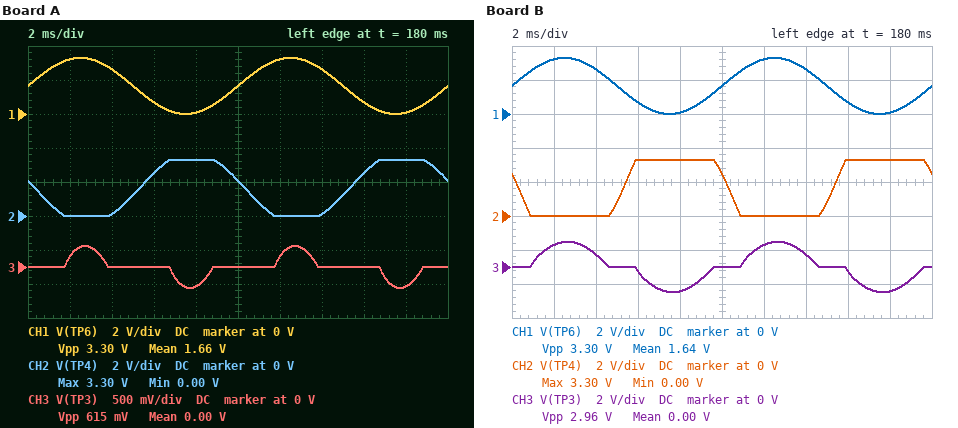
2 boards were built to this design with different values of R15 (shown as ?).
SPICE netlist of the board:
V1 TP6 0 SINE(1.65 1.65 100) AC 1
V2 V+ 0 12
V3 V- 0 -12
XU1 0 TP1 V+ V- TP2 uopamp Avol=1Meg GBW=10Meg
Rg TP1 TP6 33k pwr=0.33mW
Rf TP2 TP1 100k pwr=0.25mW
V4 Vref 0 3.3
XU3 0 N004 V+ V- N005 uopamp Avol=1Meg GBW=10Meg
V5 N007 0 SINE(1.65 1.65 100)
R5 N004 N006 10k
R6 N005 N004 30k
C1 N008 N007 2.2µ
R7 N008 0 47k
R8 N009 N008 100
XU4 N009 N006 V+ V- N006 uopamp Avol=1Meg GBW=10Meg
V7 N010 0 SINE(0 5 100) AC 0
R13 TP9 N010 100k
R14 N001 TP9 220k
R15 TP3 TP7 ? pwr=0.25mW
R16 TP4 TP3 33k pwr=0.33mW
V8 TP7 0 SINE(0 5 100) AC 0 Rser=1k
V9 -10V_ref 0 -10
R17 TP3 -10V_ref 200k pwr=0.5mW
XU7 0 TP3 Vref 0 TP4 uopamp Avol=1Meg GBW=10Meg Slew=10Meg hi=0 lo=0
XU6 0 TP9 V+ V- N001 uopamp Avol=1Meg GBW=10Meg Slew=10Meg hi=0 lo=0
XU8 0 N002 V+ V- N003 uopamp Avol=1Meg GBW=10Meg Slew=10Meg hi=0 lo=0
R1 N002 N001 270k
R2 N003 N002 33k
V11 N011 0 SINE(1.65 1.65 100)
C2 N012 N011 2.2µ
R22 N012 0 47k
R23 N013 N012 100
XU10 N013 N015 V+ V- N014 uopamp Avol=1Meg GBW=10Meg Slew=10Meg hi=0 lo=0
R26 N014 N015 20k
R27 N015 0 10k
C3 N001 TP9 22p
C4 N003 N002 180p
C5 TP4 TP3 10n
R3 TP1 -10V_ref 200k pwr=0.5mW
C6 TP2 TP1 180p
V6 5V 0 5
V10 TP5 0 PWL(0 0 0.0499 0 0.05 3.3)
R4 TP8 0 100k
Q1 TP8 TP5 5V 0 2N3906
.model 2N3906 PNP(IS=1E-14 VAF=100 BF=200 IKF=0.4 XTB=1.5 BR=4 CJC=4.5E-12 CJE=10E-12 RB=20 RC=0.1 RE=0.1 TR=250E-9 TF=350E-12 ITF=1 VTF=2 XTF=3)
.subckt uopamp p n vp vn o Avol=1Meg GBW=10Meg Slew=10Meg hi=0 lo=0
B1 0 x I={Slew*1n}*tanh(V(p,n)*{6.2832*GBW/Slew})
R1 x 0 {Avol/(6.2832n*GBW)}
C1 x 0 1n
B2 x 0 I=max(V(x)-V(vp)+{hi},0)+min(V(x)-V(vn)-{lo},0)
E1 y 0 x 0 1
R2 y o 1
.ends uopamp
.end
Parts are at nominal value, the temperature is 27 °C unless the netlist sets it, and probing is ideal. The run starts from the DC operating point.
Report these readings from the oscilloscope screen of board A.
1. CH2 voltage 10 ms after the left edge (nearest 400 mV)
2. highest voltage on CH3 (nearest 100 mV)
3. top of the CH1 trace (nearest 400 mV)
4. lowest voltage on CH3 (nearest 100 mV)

2.0 V
300 mV
3.2 V
-300 mV
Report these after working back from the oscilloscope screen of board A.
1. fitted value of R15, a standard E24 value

75 kΩ
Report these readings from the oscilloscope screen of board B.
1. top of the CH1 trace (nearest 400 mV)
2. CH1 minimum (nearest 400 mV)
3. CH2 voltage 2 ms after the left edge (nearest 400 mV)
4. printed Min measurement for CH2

3.2 V
0 V
0 V
0.00 V
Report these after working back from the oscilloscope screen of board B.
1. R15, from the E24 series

33 kΩ
